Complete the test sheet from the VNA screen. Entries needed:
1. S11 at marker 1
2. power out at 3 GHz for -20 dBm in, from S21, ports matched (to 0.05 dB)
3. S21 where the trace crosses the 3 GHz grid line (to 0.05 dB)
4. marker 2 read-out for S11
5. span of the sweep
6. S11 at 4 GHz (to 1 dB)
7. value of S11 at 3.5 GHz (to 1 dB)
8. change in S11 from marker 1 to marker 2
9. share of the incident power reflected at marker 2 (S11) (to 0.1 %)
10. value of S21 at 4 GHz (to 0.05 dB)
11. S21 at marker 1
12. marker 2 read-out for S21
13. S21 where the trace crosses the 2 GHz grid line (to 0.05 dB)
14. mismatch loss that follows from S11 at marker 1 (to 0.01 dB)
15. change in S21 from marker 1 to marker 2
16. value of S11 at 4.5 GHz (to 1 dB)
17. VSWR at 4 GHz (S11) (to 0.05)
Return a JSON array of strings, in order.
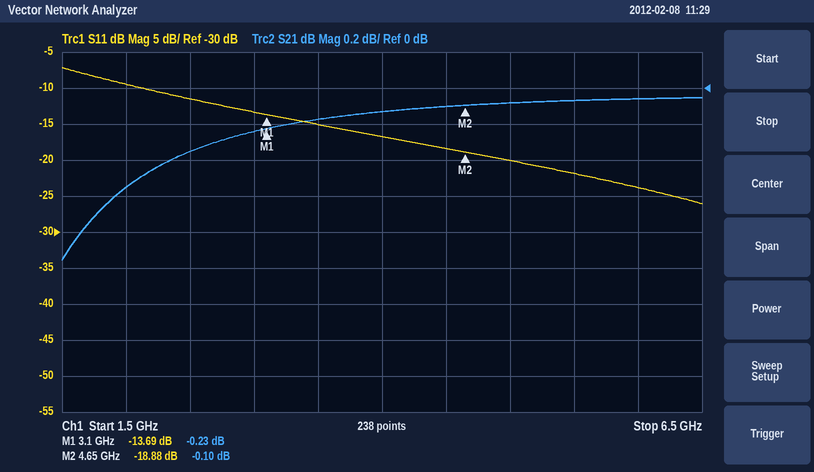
["-13.69 dB", "-20.25 dBm", "-0.25 dB", "-18.88 dB", "5 GHz", "-17 dB", "-15 dB", "-5.19 dB", "1.3 %", "-0.15 dB", "-0.23 dB", "-0.10 dB", "-0.55 dB", "0.19 dB", "0.13 dB", "-18 dB", "1.35"]
